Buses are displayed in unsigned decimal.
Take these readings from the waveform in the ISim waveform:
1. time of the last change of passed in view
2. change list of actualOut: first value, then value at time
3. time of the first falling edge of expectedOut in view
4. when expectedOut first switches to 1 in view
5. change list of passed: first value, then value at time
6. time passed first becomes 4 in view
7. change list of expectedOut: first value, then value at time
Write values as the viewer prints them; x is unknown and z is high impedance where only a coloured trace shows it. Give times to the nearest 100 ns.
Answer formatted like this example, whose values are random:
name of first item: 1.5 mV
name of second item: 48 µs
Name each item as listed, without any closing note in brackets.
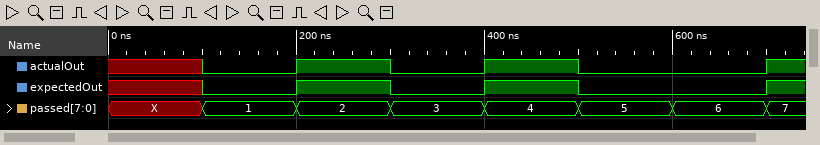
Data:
time of the last change of passed in view: 700 ns
change list of actualOut: first value, then value at time: x, 0 at 100 ns, 1 at 200 ns, 0 at 300 ns, 1 at 400 ns, 0 at 500 ns, 1 at 700 ns
time of the first falling edge of expectedOut in view: 300 ns
when expectedOut first switches to 1 in view: 200 ns
change list of passed: first value, then value at time: X, 1 at 100 ns, 2 at 200 ns, 3 at 300 ns, 4 at 400 ns, 5 at 500 ns, 6 at 600 ns, 7 at 700 ns
time passed first becomes 4 in view: 400 ns
change list of expectedOut: first value, then value at time: x, 0 at 100 ns, 1 at 200 ns, 0 at 300 ns, 1 at 400 ns, 0 at 500 ns, 1 at 700 ns
